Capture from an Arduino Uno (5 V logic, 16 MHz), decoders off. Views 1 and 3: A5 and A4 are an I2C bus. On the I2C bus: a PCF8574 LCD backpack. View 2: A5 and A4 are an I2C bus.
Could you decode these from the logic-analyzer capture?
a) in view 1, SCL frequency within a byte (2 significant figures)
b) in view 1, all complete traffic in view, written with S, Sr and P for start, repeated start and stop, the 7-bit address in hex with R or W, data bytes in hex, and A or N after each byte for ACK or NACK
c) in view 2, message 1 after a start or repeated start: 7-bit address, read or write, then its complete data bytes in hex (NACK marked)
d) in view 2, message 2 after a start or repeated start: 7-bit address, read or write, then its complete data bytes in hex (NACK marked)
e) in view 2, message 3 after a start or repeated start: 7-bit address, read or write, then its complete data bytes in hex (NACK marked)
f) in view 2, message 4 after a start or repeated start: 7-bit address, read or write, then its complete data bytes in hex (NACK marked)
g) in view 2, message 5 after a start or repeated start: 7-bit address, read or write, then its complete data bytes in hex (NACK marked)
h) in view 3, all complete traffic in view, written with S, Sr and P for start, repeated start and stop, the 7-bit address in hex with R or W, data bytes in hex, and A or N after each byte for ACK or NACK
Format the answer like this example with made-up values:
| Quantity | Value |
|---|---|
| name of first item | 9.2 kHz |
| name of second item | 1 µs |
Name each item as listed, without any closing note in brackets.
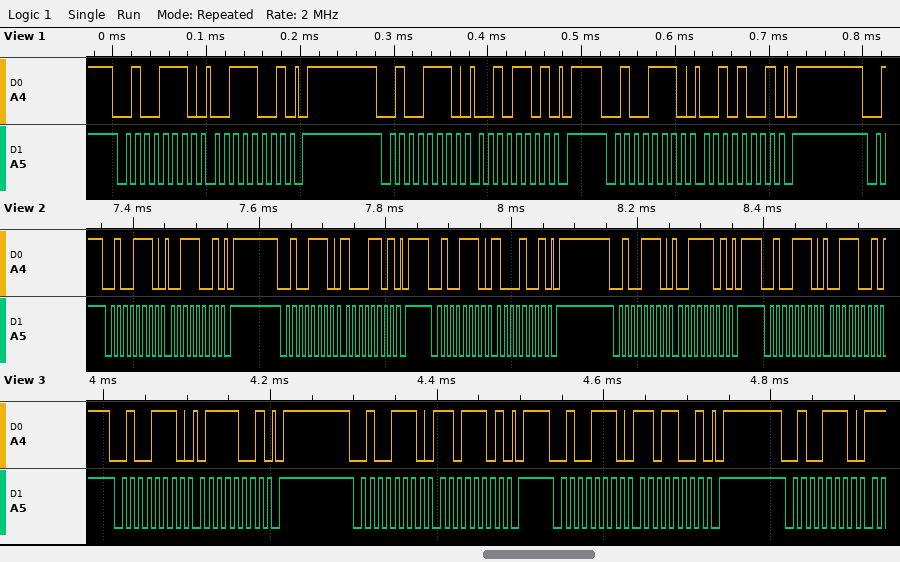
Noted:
| Quantity | Value |
|---|---|
| in view 1, SCL frequency within a byte | 100 kHz |
| in view 1, all complete traffic in view, written with S, Sr and P for start, repeated start and stop, the 7-bit address in hex with R or W, data bytes in hex, and A or N after each byte for ACK or NACK | S 27W A 39 A P S 27W A 2D A P S 27W A 29 A P |
| in view 2, message 1 after a start or repeated start: 7-bit address, read or write, then its complete data bytes in hex | 0x27 write: 39 |
| in view 2, message 2 after a start or repeated start: 7-bit address, read or write, then its complete data bytes in hex | 0x27 write: 8D |
| in view 2, message 3 after a start or repeated start: 7-bit address, read or write, then its complete data bytes in hex | 0x27 write: 89 |
| in view 2, message 4 after a start or repeated start: 7-bit address, read or write, then its complete data bytes in hex | 0x27 write: 3D |
| in view 2, message 5 after a start or repeated start: 7-bit address, read or write, then its complete data bytes in hex | 0x27 write: 39 |
| in view 3, all complete traffic in view, written with S, Sr and P for start, repeated start and stop, the 7-bit address in hex with R or W, data bytes in hex, and A or N after each byte for ACK or NACK | S 27W A 79 A P S 27W A DD A P S 27W A D9 A P S 27W A |
